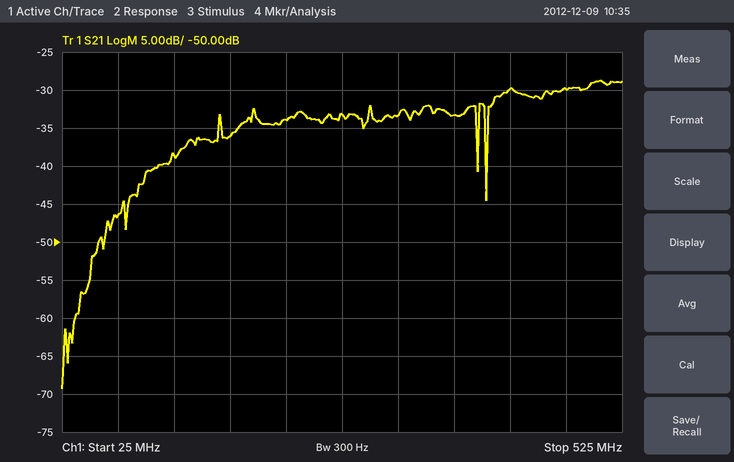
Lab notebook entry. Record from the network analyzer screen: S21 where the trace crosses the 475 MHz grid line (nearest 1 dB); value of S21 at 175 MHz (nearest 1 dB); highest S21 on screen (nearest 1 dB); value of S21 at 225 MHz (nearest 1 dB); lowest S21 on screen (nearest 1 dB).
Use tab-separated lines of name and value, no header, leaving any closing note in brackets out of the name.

S21 where the trace crosses the 475 MHz grid line	-30 dB
value of S21 at 175 MHz	-36 dB
highest S21 on screen	-29 dB
value of S21 at 225 MHz	-34 dB
lowest S21 on screen	-69 dB
